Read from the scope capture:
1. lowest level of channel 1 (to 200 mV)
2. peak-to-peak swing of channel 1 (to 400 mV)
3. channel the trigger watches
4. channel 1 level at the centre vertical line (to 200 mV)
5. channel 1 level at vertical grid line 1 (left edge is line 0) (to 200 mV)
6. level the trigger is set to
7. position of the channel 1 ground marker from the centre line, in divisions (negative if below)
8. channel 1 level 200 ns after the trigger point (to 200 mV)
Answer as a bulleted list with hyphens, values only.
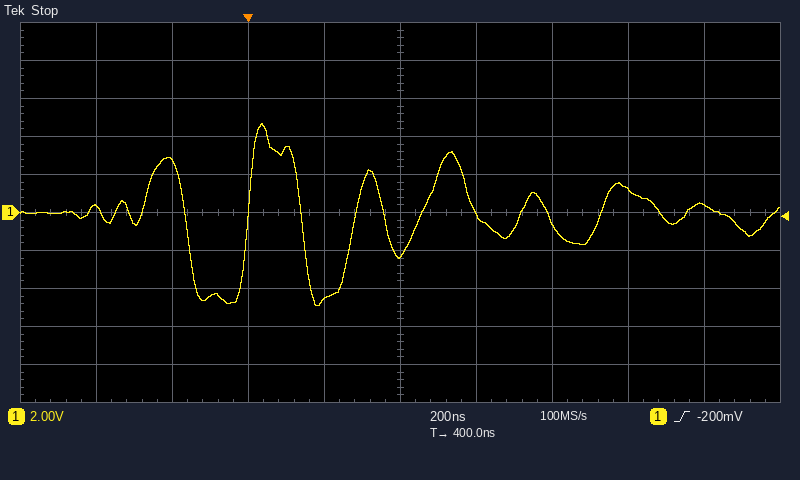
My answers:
- -4.8 V
- 9.6 V
- channel 1
- -2.2 V
- 200 mV
- -200 mV
- 0.0 div
- -4.6 V
